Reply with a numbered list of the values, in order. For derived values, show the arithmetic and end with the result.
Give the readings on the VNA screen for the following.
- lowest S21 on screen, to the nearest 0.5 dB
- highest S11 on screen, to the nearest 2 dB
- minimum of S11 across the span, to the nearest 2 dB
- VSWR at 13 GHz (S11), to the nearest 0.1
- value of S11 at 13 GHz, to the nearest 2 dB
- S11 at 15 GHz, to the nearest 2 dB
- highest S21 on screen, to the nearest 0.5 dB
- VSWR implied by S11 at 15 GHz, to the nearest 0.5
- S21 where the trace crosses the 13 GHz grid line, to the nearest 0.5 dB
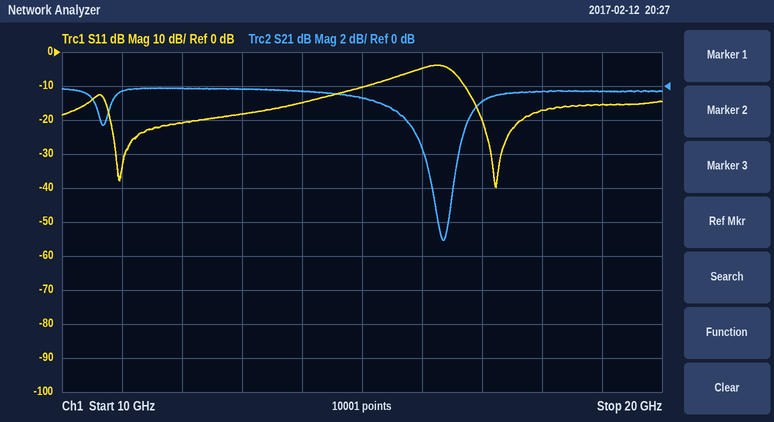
1. -9.0 dB
2. -4 dB
3. -40 dB
4. |Γ| = 10^(-18/20) = 0.1259; VSWR = (1 + 0.1259)/(1 − 0.1259) ≈ 1.3
5. -18 dB
6. -10 dB
7. 0.0 dB
8. |Γ| = 10^(-10/20) = 0.3162; VSWR = (1 + 0.3162)/(1 − 0.3162) ≈ 1.92, so 2.0 to the nearest 0.5
9. 0.0 dB
